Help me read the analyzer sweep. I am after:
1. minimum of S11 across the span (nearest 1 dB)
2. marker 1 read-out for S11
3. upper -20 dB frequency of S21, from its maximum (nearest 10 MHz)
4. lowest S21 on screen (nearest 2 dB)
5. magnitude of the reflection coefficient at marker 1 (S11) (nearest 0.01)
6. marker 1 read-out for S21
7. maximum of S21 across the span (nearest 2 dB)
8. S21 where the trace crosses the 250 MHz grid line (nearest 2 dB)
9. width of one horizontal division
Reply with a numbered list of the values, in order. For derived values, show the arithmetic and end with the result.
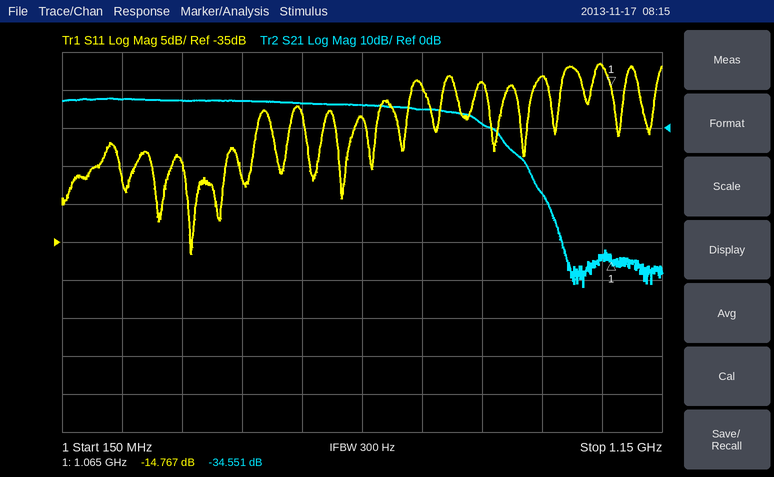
1. -37 dB
2. -14.767 dB
3. 930 MHz
4. -42 dB
5. 10^(-14.767/20) ≈ 0.18
6. -34.551 dB
7. 8 dB
8. 8 dB
9. 100 MHz
